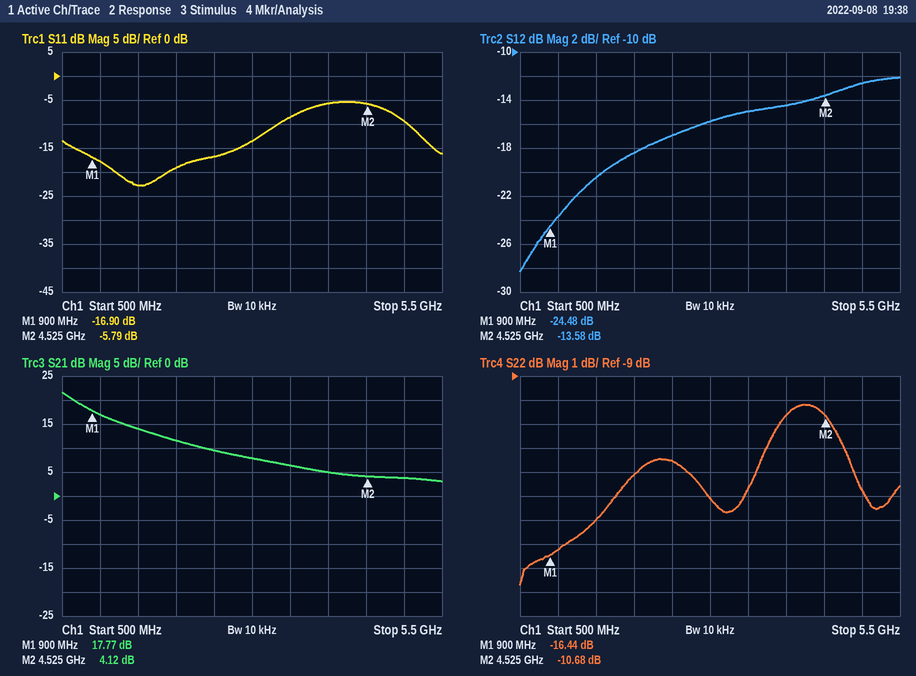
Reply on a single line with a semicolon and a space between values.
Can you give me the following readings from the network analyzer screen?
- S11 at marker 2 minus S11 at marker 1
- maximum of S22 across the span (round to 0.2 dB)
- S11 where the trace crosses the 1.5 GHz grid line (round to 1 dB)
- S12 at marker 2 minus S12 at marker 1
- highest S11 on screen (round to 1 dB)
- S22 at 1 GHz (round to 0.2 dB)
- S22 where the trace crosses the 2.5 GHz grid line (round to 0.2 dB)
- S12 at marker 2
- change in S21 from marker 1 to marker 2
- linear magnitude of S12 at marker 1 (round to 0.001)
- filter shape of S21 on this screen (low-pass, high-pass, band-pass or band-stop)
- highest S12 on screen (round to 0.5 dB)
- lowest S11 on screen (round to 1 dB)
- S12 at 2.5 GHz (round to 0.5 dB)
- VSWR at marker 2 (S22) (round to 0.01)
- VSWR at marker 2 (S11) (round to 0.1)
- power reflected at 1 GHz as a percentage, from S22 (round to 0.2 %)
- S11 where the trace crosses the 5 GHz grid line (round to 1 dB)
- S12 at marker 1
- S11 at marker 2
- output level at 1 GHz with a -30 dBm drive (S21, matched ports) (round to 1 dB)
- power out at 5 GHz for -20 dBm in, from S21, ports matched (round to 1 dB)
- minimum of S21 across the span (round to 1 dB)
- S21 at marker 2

11.11 dB; -10.2 dB; -23 dB; 10.90 dB; -5 dB; -16.2 dB; -12.6 dB; -13.58 dB; -13.65 dB; 0.060; low-pass; -12.0 dB; -23 dB; -17.0 dB; 1.83; 3.1; 2.4 %; -9 dB; -24.48 dB; -5.79 dB; -13 dBm; -16 dBm; 3 dB; 4.12 dB
